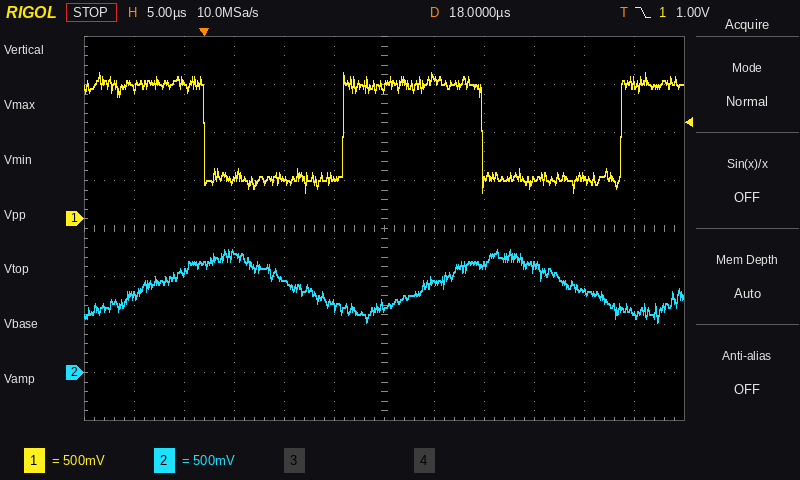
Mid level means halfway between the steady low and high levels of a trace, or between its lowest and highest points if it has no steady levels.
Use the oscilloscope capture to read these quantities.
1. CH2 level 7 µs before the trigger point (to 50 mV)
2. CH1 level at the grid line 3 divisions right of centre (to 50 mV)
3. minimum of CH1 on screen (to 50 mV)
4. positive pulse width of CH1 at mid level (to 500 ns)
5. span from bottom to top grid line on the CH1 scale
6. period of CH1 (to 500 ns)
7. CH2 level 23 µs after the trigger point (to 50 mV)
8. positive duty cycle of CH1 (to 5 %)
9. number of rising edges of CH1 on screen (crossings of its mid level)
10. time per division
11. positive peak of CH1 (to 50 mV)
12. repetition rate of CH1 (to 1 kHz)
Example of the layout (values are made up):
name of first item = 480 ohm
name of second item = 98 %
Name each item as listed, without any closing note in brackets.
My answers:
CH2 level 7 µs before the trigger point = 800 mV
CH1 level at the grid line 3 divisions right of centre = 400 mV
minimum of CH1 on screen = 300 mV
positive pulse width of CH1 at mid level = 14.0 µs
span from bottom to top grid line on the CH1 scale = 4 V
period of CH1 = 28.0 µs
CH2 level 23 µs after the trigger point = 950 mV
positive duty cycle of CH1 = 50 %
number of rising edges of CH1 on screen = 2
time per division = 5 µs
positive peak of CH1 = 1.50 V
repetition rate of CH1 = 36 kHz
